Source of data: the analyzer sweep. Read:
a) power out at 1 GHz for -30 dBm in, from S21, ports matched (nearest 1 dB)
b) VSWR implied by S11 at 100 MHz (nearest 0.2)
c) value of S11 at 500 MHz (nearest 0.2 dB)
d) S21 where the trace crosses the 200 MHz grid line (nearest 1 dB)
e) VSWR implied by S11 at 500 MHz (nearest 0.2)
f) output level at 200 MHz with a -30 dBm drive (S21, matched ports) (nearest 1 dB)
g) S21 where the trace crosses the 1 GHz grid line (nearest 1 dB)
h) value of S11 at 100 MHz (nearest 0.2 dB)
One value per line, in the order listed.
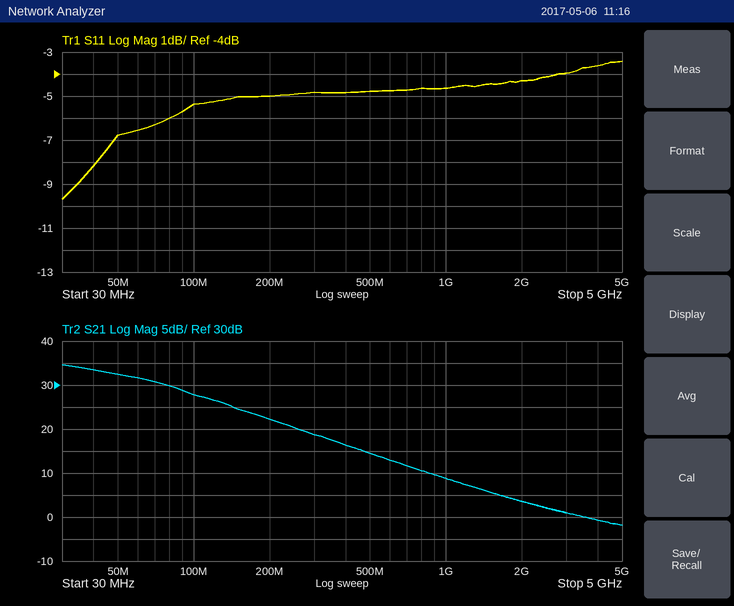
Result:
-21 dBm
3.4
-4.8 dB
22 dB
3.8
-8 dBm
9 dB
-5.4 dB
